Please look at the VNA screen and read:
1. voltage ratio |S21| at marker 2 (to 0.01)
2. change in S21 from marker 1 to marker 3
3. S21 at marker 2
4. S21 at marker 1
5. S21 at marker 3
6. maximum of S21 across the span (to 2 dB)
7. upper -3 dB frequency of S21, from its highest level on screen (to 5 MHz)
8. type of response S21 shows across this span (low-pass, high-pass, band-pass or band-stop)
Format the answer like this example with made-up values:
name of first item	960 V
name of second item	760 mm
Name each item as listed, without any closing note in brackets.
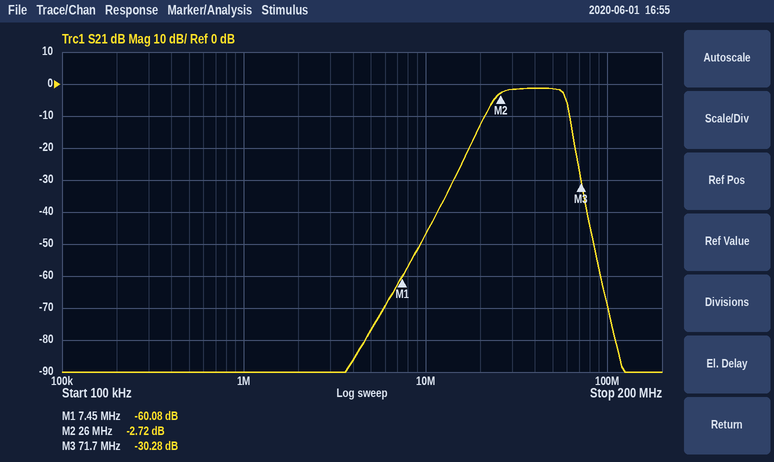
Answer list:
voltage ratio |S21| at marker 2	0.73
change in S21 from marker 1 to marker 3	29.80 dB
S21 at marker 2	-2.72 dB
S21 at marker 1	-60.08 dB
S21 at marker 3	-30.28 dB
maximum of S21 across the span	-2 dB
upper -3 dB frequency of S21, from its highest level on screen	60 MHz
type of response S21 shows across this span	band-pass
